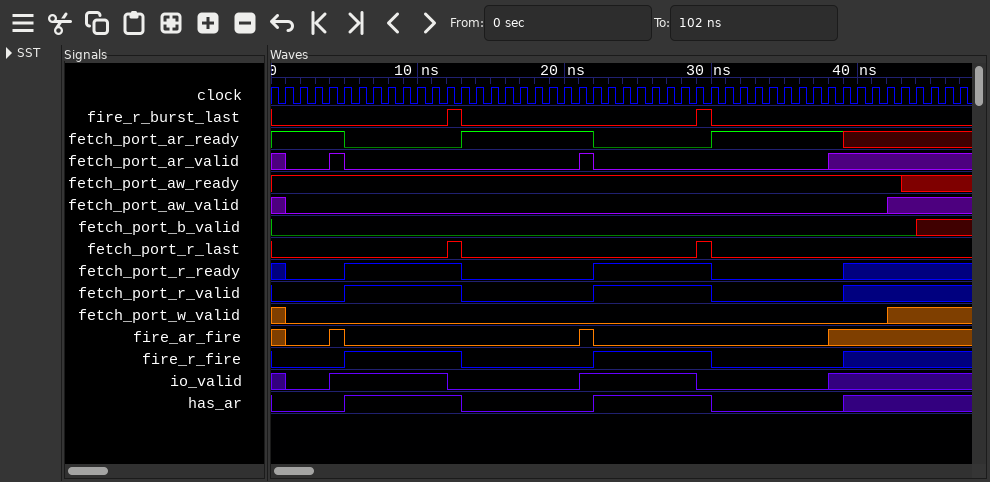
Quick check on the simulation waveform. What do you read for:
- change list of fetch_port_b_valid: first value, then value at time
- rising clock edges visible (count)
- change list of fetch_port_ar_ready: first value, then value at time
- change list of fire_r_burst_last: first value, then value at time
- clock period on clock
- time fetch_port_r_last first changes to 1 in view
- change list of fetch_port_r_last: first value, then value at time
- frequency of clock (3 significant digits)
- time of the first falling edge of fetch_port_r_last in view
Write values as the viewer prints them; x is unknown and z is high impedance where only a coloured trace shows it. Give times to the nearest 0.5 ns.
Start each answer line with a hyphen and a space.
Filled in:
- 0, x at 44 ns
- 47
- 1, 0 at 5 ns, 1 at 13 ns, 0 at 22 ns, 1 at 30 ns, x at 39 ns
- 0, 1 at 12 ns, 0 at 13 ns, 1 at 29 ns, 0 at 30 ns
- 1 ns
- 12 ns
- 0, 1 at 12 ns, 0 at 13 ns, 1 at 29 ns, 0 at 30 ns
- 1.00 GHz
- 13 ns
